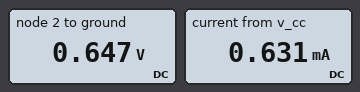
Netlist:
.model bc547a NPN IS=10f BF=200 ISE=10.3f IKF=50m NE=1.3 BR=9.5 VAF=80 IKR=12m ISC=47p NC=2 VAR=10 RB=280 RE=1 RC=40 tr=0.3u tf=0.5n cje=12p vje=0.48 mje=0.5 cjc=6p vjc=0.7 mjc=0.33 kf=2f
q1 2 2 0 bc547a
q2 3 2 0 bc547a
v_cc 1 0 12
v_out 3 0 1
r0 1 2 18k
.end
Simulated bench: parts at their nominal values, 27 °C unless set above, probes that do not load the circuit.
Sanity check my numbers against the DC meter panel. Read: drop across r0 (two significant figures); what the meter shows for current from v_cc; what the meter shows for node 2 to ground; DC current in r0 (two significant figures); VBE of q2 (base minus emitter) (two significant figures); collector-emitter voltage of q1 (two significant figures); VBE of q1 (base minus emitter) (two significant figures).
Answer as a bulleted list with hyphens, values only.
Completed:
- 11 V
- 0.631 mA
- 0.647 V
- 630 µA
- 650 mV
- 650 mV
- 650 mV
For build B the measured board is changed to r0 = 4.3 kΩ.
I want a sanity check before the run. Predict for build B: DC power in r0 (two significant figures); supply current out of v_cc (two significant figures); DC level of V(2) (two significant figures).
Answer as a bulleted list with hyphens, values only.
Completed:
- 30 mW
- 2.6 mA
- 690 mV
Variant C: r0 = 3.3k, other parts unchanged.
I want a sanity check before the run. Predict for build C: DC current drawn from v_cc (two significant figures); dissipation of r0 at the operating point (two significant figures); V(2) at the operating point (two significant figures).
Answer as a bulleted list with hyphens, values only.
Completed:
- 3.4 mA
- 39 mW
- 700 mV
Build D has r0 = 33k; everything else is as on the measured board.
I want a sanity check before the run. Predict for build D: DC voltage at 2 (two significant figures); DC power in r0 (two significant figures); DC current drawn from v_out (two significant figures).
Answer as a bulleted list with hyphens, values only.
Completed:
- 630 mV
- 3.9 mW
- 340 µA
